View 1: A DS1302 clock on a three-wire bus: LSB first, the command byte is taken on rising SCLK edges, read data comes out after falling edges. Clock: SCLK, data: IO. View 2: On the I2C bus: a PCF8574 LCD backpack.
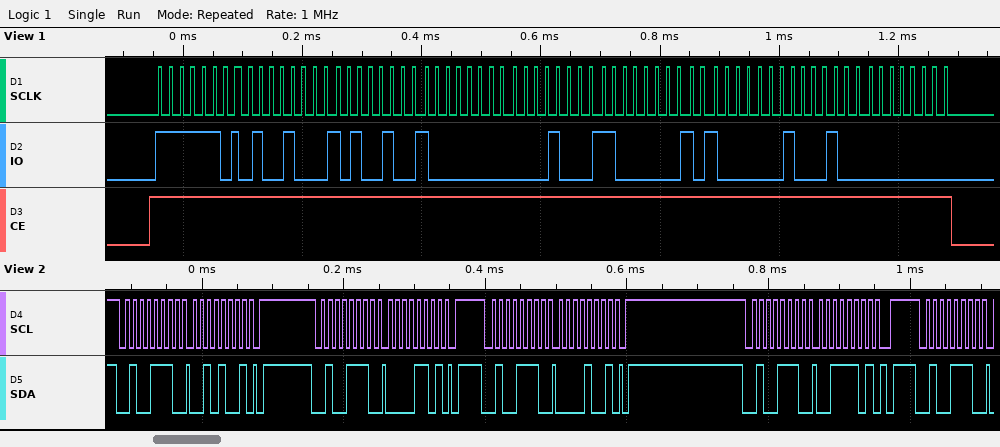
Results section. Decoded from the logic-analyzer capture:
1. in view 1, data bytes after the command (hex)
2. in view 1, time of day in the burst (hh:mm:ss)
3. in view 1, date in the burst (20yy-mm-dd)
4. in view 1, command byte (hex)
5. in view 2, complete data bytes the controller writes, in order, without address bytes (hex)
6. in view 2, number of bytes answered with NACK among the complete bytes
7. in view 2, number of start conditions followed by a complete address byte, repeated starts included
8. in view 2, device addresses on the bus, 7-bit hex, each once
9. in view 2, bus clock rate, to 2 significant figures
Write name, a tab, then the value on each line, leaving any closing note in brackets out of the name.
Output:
in view 1, data bytes after the command	12 25 01 10 03 05 22 00
in view 1, time of day in the burst	01:25:12
in view 1, date in the burst	2022-03-10
in view 1, command byte	0xBF
in view 2, complete data bytes the controller writes, in order, without address bytes	29 0D 09 3D
in view 2, number of bytes answered with NACK among the complete bytes	0
in view 2, number of start conditions followed by a complete address byte, repeated starts included	5
in view 2, device addresses on the bus, 7-bit hex, each once	0x27
in view 2, bus clock rate, to 2 significant figures	100 kHz
